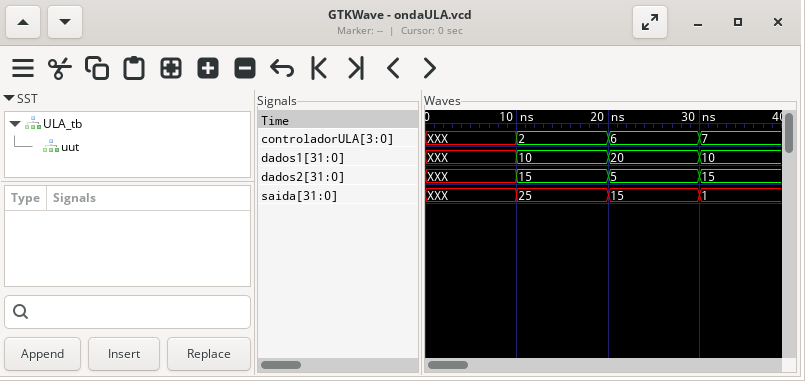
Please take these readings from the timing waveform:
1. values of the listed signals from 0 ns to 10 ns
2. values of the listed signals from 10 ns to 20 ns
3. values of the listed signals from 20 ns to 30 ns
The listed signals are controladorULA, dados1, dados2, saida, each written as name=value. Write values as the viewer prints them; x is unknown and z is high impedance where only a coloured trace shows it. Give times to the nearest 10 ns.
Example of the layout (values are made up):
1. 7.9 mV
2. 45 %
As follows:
1. controladorULA=XXX, dados1=XXX, dados2=XXX, saida=XXX
2. controladorULA=2, dados1=10, dados2=15, saida=25
3. controladorULA=6, dados1=20, dados2=5, saida=15
